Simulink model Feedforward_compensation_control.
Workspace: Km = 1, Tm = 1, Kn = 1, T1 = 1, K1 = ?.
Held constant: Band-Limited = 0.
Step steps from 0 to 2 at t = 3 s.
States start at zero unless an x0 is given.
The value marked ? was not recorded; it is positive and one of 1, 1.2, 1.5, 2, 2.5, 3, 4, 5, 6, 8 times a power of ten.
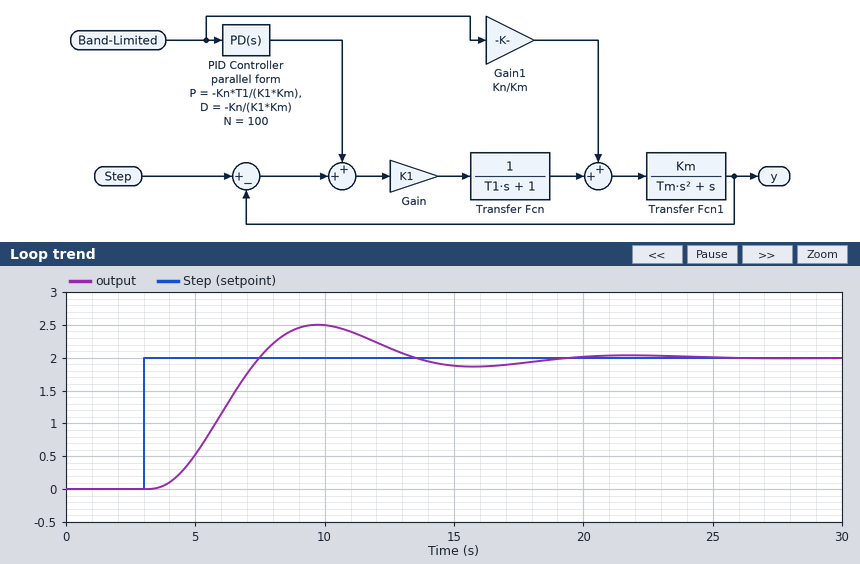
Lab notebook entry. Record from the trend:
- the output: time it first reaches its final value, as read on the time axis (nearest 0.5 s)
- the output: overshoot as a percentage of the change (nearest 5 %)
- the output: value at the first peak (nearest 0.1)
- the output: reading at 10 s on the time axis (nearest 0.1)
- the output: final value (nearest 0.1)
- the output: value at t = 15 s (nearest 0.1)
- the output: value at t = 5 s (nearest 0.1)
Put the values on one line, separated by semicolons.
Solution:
7.5 s; 25 %; 2.5; 2.5; 2.0; 1.9; 0.5
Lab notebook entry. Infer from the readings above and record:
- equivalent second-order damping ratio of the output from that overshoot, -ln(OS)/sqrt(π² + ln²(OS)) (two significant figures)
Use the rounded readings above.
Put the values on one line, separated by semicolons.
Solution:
0.40
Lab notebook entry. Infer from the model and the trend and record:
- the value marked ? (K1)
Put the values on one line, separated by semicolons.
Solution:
0.5
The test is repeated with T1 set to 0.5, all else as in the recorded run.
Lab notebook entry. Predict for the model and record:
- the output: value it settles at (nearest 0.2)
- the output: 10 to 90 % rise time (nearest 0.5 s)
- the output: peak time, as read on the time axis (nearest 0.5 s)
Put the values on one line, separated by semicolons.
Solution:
2.0; 2.5 s; 9.0 s
